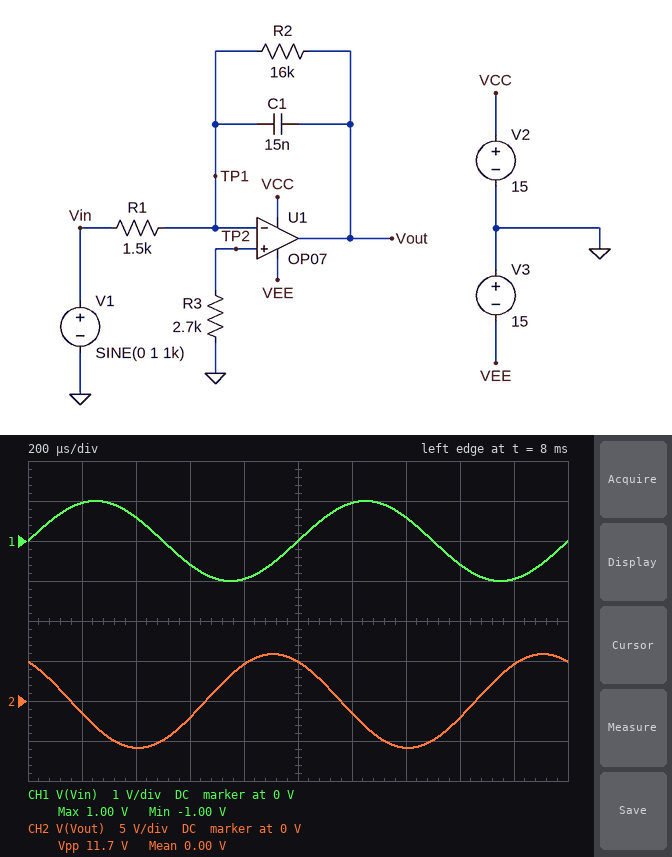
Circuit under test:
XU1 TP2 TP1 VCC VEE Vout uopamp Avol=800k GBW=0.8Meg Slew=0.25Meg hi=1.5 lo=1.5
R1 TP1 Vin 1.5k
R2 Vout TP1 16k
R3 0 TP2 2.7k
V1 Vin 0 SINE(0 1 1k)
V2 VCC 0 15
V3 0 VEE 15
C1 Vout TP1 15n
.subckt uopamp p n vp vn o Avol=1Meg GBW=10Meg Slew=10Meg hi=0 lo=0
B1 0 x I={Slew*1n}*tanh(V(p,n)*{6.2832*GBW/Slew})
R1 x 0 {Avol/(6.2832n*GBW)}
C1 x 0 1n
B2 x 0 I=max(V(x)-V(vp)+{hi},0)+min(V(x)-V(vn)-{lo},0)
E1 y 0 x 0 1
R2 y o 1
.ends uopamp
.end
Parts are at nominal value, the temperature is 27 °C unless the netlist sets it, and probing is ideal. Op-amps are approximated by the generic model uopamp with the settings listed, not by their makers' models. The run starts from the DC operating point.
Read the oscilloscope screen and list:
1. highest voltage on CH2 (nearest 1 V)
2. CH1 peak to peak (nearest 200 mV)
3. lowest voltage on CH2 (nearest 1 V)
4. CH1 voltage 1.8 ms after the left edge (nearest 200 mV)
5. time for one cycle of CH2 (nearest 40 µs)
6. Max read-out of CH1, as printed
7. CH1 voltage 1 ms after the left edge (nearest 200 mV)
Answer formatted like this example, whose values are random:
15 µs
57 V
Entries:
6 V
2.0 V
-6 V
-1.0 V
1.00 ms
1.00 V
0 V
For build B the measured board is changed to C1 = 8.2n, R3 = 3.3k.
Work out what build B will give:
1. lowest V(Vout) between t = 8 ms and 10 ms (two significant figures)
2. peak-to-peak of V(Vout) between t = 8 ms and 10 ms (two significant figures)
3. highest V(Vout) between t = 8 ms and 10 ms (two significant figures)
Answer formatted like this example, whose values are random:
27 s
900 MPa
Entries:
-8.2 V
16 V
8.2 V
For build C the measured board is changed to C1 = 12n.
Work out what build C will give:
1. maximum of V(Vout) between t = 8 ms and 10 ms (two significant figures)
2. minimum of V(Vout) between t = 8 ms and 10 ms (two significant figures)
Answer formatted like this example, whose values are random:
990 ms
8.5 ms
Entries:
6.8 V
-6.8 V
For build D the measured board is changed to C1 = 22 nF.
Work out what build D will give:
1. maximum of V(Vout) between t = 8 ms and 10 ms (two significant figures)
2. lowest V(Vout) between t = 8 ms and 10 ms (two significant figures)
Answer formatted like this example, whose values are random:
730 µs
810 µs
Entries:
4.4 V
-4.4 V
